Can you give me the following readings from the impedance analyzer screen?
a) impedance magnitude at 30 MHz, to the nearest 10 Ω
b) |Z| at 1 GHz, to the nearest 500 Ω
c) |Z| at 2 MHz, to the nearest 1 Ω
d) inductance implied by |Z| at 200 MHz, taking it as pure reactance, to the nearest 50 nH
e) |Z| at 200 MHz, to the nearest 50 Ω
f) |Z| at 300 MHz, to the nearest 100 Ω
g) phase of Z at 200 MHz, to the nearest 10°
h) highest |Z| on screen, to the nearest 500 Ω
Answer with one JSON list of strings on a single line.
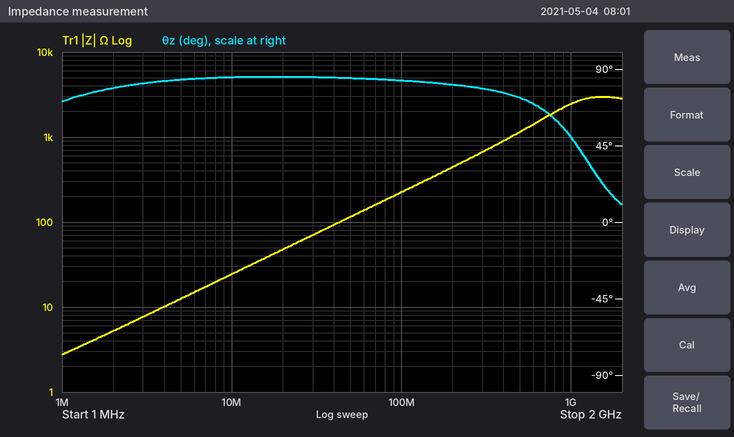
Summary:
["70 Ω", "2.5 kΩ", "5 Ω", "350 nH", "450 Ω", "700 Ω", "80°", "3.0 kΩ"]
